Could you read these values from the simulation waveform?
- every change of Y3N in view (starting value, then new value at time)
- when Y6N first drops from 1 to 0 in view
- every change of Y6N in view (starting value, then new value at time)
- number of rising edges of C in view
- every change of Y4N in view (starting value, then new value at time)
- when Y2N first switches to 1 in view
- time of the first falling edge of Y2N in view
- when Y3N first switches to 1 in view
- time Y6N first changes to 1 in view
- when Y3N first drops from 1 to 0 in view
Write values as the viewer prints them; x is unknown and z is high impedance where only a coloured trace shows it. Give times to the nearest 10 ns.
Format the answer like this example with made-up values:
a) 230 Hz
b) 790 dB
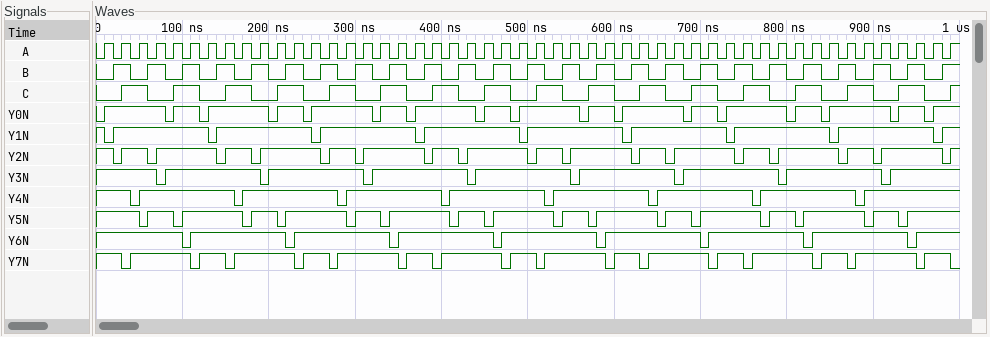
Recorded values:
a) 1, 0 at 70 ns, 1 at 80 ns, 0 at 190 ns, 1 at 200 ns, 0 at 310 ns, 1 at 320 ns, 0 at 430 ns, 1 at 440 ns, 0 at 550 ns, 1 at 560 ns, 0 at 670 ns, 1 at 680 ns, 0 at 790 ns, 1 at 800 ns, 0 at 910 ns, 1 at 920 ns
b) 100 ns
c) 1, 0 at 100 ns, 1 at 110 ns, 0 at 220 ns, 1 at 230 ns, 0 at 340 ns, 1 at 350 ns, 0 at 460 ns, 1 at 470 ns, 0 at 580 ns, 1 at 590 ns, 0 at 700 ns, 1 at 710 ns, 0 at 820 ns, 1 at 830 ns, 0 at 940 ns, 1 at 950 ns
d) 17
e) 1, 0 at 40 ns, 1 at 50 ns, 0 at 160 ns, 1 at 170 ns, 0 at 280 ns, 1 at 290 ns, 0 at 400 ns, 1 at 410 ns, 0 at 520 ns, 1 at 530 ns, 0 at 640 ns, 1 at 650 ns, 0 at 760 ns, 1 at 770 ns, 0 at 880 ns, 1 at 890 ns
f) 30 ns
g) 20 ns
h) 80 ns
i) 110 ns
j) 70 ns
